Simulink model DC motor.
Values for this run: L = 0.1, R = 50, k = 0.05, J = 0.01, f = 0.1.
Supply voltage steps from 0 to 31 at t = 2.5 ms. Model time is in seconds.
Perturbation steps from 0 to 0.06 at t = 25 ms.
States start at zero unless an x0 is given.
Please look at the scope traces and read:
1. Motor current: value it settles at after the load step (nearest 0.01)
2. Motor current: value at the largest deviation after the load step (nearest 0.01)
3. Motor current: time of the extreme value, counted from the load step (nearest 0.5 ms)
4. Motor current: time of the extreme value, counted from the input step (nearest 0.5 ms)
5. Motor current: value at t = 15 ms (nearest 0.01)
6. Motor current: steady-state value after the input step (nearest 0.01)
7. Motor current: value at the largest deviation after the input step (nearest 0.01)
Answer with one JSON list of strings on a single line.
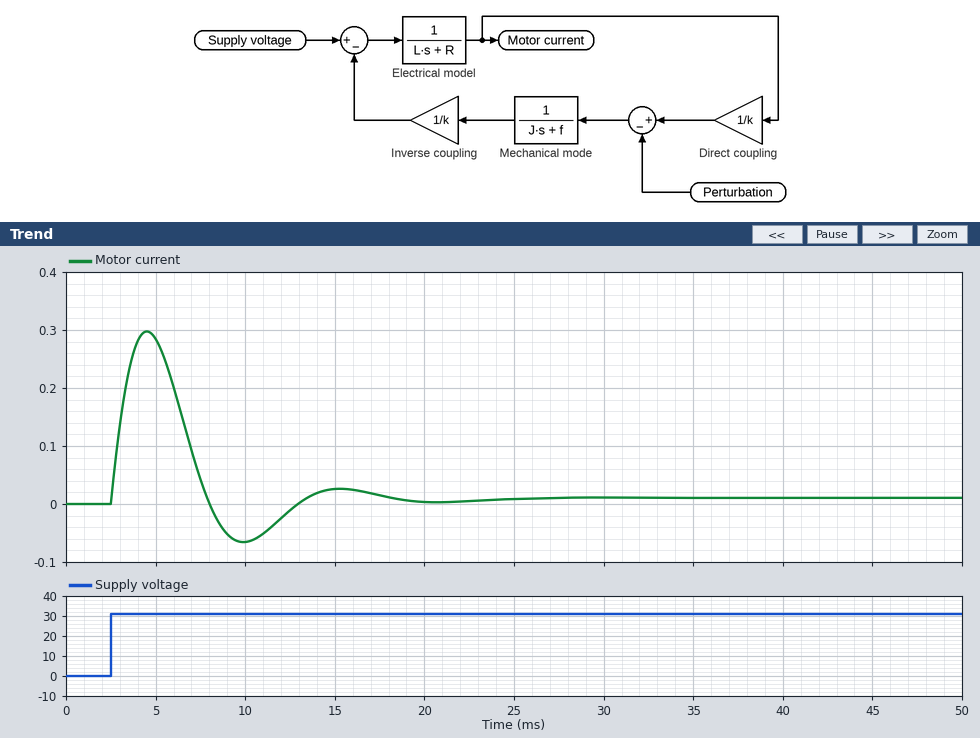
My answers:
["0.01", "0.01", "4.5 ms", "2.0 ms", "0.03", "0.01", "0.30"]
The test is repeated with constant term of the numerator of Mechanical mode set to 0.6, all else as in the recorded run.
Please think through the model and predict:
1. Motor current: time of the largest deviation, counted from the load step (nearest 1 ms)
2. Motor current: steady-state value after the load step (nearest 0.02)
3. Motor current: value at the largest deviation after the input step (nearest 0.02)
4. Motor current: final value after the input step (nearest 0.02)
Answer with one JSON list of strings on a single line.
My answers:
["8 ms", "0.02", "0.34", "0.02"]
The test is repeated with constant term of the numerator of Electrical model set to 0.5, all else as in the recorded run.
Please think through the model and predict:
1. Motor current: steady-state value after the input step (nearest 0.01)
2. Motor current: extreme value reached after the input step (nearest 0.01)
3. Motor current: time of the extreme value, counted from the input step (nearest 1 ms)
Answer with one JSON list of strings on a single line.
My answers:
["0.01", "0.18", "3 ms"]
